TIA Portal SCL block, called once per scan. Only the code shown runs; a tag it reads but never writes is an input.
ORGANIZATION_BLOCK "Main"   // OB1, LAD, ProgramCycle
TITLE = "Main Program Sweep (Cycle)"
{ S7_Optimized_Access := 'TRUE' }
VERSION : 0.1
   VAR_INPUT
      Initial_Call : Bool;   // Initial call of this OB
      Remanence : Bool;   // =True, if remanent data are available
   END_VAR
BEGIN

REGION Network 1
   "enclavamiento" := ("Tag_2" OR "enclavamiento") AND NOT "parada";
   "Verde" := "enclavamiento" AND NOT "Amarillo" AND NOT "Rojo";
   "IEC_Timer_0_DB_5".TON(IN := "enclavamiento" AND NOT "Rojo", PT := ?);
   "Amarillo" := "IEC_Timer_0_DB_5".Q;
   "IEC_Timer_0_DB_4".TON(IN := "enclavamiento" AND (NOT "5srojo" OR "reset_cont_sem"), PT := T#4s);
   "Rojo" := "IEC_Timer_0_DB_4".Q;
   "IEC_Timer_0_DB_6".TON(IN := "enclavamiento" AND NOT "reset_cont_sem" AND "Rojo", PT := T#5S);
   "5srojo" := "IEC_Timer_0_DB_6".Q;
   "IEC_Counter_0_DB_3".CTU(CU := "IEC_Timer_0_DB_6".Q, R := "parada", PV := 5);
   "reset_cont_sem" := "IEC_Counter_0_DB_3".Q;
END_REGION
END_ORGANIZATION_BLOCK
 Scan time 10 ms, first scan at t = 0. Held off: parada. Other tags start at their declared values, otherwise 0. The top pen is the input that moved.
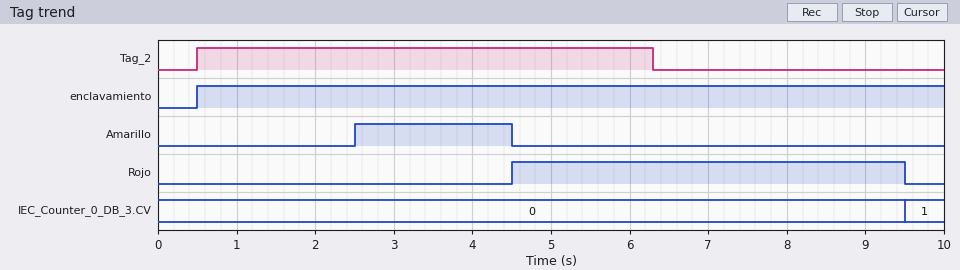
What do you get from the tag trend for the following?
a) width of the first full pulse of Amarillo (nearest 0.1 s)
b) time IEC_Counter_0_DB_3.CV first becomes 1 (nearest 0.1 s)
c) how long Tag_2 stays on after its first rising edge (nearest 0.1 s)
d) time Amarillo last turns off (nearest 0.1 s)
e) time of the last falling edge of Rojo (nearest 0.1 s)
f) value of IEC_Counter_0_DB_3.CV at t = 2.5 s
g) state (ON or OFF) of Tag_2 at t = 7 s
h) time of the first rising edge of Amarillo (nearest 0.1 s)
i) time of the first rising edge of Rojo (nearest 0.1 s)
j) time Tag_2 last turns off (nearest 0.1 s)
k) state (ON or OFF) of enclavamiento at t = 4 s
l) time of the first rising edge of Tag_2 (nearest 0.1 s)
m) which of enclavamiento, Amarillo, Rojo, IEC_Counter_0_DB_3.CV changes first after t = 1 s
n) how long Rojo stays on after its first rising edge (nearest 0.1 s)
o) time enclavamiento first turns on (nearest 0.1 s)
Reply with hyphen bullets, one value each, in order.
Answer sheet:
- 2.0 s
- 9.5 s
- 5.8 s
- 4.5 s
- 9.5 s
- 0
- OFF
- 2.5 s
- 4.5 s
- 6.3 s
- ON
- 0.5 s
- Amarillo
- 5.0 s
- 0.5 s
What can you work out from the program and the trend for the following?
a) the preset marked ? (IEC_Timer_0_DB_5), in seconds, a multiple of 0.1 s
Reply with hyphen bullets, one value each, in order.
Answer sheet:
- 2.0 s
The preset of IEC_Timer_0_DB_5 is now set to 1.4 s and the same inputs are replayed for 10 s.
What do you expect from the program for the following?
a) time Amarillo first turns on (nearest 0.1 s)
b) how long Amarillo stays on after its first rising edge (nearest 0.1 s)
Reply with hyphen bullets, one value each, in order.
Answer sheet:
- 1.9 s
- 2.6 s
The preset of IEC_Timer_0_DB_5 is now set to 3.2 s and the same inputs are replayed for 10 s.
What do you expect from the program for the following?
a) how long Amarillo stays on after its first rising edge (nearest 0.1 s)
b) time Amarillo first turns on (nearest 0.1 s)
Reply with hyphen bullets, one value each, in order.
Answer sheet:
- 0.8 s
- 3.7 s
